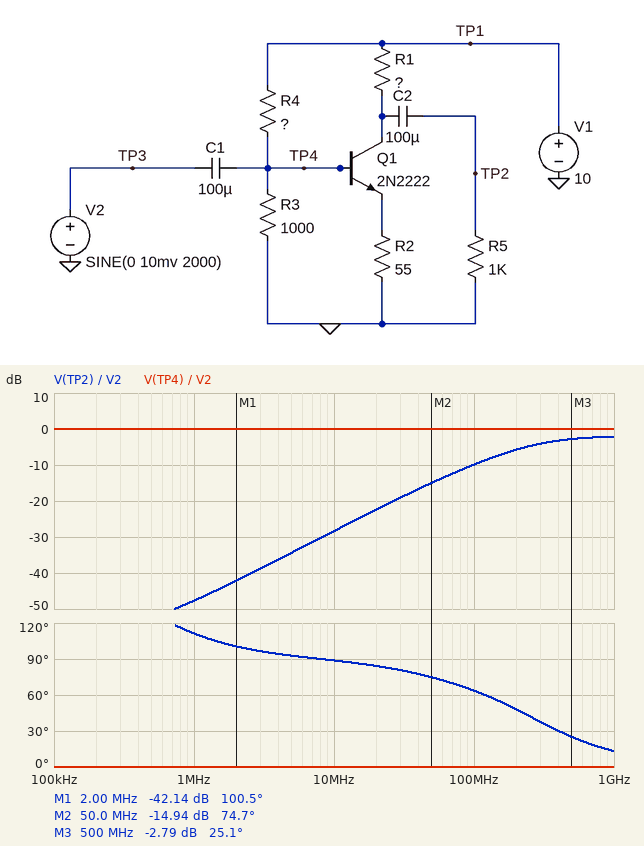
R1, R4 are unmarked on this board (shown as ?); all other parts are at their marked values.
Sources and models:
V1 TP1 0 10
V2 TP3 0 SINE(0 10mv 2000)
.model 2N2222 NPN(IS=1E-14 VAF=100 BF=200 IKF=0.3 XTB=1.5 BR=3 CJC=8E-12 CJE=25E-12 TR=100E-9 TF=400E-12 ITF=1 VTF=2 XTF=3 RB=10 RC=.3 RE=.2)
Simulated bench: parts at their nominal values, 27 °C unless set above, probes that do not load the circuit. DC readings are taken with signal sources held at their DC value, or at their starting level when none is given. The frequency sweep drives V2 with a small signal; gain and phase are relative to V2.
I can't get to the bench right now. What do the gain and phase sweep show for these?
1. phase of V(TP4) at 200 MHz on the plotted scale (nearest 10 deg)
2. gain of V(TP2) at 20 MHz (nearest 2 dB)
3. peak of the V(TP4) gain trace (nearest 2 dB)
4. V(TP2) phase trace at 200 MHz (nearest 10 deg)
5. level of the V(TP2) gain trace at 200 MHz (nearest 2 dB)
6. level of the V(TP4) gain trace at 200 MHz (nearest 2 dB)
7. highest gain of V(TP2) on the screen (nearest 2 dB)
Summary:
0 deg
-22 dB
0 dB
50 deg
-6 dB
0 dB
-2 dB
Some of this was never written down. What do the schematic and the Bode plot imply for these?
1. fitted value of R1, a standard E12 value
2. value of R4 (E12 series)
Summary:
220 Ω
22 kΩ
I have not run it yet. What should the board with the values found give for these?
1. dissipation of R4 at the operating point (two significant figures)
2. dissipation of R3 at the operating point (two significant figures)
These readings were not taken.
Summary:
4.2 mW
190 µW
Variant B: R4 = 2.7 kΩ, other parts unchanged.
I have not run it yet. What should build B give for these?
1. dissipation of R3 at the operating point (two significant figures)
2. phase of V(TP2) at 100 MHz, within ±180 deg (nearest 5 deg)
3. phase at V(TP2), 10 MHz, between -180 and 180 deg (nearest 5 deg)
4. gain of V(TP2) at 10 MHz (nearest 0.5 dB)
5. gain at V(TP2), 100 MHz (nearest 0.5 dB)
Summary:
6.6 mW
105 deg
170 deg
10.0 dB
7.0 dB
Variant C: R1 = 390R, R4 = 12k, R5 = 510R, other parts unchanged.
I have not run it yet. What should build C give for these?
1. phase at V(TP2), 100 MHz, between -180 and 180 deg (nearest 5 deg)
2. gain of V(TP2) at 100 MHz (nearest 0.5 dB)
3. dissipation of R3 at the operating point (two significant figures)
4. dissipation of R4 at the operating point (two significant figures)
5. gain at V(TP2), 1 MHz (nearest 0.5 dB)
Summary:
115 deg
8.0 dB
580 µW
7.1 mW
10.0 dB
